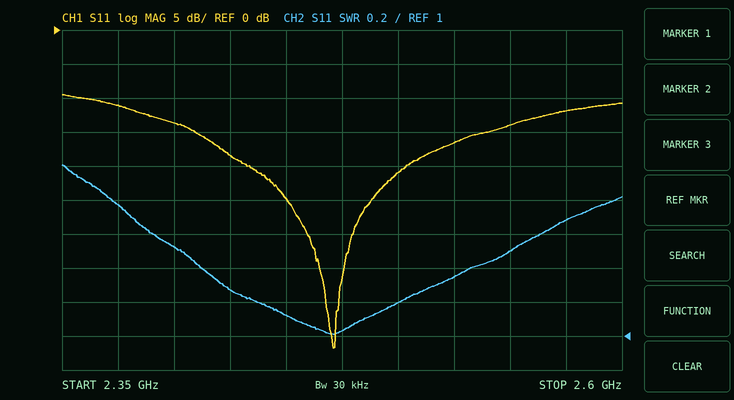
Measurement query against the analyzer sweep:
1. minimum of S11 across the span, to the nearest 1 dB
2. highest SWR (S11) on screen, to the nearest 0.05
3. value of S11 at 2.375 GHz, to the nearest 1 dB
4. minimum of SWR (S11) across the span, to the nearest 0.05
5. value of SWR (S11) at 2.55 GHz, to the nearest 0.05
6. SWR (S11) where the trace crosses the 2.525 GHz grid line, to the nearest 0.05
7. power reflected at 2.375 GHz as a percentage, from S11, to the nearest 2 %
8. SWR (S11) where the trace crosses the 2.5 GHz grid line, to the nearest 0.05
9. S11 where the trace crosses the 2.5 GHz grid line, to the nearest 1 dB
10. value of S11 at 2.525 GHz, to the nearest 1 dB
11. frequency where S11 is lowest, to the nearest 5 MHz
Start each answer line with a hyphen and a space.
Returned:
- -47 dB
- 2.00
- -11 dB
- 1.00
- 1.50
- 1.35
- 8 %
- 1.20
- -21 dB
- -17 dB
- 2.470 GHz
